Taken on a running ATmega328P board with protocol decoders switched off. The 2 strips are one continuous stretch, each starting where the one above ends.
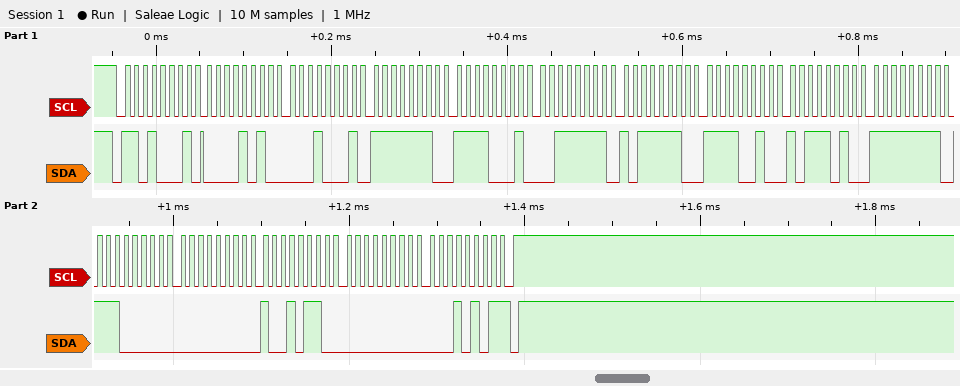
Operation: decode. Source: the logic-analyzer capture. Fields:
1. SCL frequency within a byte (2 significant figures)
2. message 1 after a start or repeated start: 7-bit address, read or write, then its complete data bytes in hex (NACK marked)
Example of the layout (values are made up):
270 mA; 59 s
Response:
100 kHz; 0x68 read: 0A 11 FE F1 3F BE F2 BA FF E0 00 96 00 15 NACK
